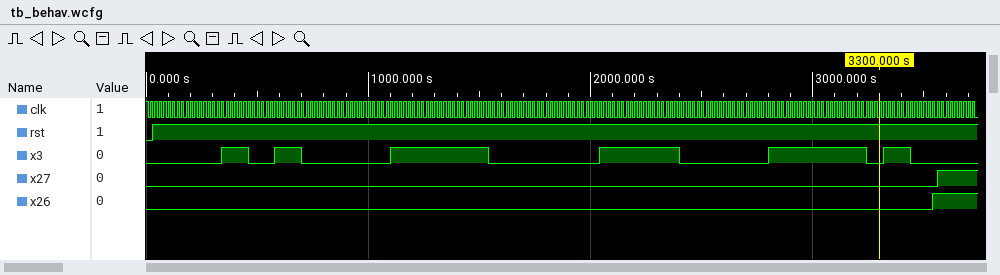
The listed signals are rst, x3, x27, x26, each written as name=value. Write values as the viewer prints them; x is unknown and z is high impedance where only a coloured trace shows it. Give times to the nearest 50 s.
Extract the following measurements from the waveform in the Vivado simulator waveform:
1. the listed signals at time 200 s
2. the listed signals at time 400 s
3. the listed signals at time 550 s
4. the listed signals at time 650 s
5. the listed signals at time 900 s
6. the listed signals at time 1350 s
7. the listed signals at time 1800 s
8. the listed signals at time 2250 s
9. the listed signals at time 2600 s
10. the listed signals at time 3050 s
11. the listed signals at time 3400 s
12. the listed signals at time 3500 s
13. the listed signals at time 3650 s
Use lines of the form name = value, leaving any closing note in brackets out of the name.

the listed signals at time 200 s = rst=1, x3=0, x27=0, x26=0
the listed signals at time 400 s = rst=1, x3=1, x27=0, x26=0
the listed signals at time 550 s = rst=1, x3=0, x27=0, x26=0
the listed signals at time 650 s = rst=1, x3=1, x27=0, x26=0
the listed signals at time 900 s = rst=1, x3=0, x27=0, x26=0
the listed signals at time 1350 s = rst=1, x3=1, x27=0, x26=0
the listed signals at time 1800 s = rst=1, x3=0, x27=0, x26=0
the listed signals at time 2250 s = rst=1, x3=1, x27=0, x26=0
the listed signals at time 2600 s = rst=1, x3=0, x27=0, x26=0
the listed signals at time 3050 s = rst=1, x3=1, x27=0, x26=0
the listed signals at time 3400 s = rst=1, x3=1, x27=0, x26=0
the listed signals at time 3500 s = rst=1, x3=0, x27=0, x26=0
the listed signals at time 3650 s = rst=1, x3=0, x27=1, x26=1
